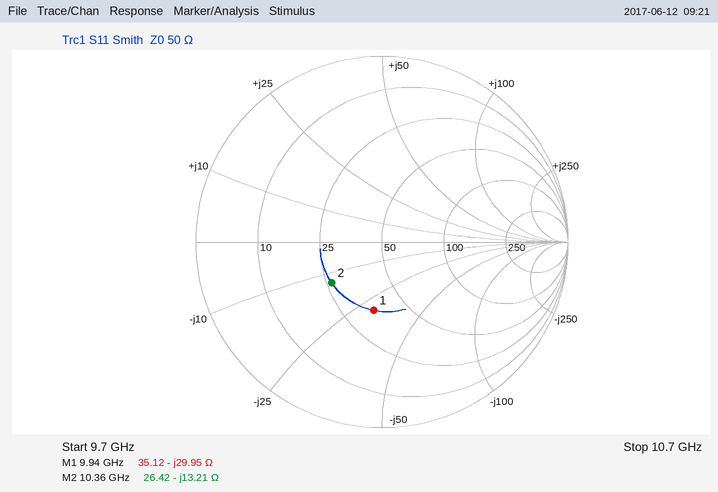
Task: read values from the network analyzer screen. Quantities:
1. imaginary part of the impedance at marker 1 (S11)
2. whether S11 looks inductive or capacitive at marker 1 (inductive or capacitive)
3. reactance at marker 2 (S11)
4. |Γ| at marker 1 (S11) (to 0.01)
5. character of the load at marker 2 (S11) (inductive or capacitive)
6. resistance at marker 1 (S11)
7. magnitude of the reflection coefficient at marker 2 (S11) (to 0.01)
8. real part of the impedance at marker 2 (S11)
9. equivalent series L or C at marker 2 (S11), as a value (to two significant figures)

-29.95 Ω
capacitive
-13.21 Ω
0.37
capacitive
35.12 Ω
0.35
26.42 Ω
1.2 pF
